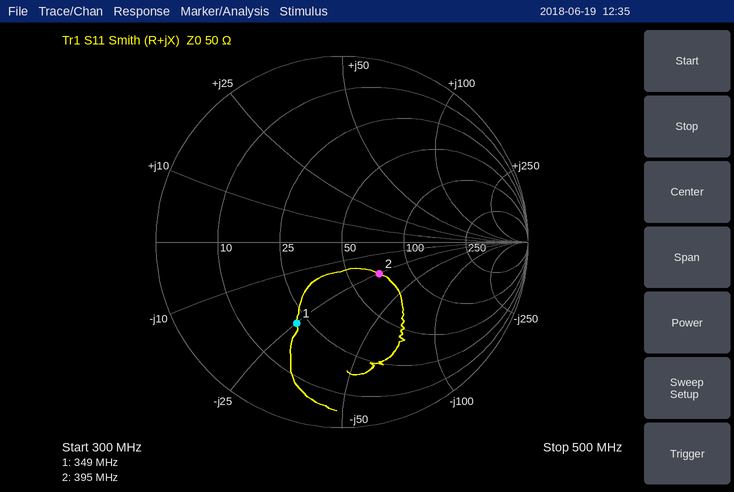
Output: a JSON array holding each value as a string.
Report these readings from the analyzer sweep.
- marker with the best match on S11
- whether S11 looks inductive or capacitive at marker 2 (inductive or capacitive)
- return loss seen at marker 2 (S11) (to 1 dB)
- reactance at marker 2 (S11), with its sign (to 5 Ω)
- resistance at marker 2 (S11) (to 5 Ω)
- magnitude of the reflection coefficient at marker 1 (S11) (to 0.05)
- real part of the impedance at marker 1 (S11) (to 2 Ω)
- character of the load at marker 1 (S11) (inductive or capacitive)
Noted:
["marker 2", "capacitive", "12 dB", "-25 Ω", "70 Ω", "0.50", "22 Ω", "capacitive"]
